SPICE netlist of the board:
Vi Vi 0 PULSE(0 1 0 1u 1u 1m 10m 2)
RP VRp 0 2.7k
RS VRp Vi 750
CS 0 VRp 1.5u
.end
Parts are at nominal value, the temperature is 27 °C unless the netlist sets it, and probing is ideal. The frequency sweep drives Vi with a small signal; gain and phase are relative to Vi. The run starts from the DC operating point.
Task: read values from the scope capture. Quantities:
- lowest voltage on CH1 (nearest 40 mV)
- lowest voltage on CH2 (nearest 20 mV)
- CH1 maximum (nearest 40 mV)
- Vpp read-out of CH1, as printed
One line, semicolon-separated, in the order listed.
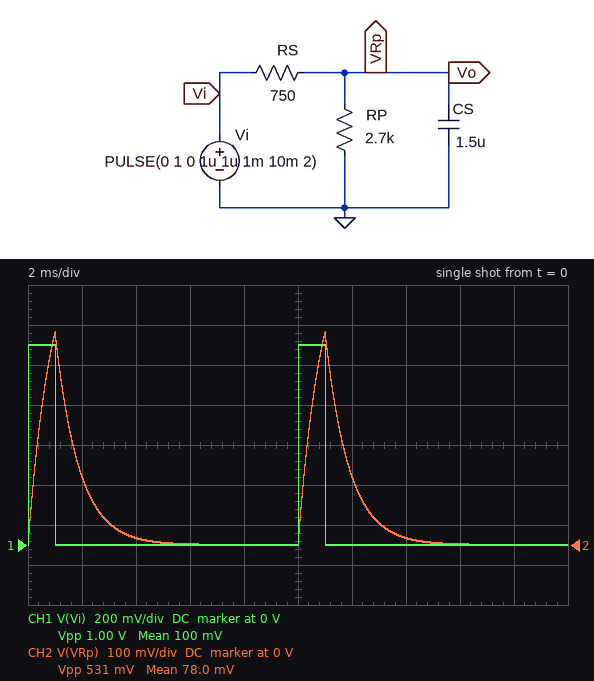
0 V; 0 V; 1.00 V; 1.00 V
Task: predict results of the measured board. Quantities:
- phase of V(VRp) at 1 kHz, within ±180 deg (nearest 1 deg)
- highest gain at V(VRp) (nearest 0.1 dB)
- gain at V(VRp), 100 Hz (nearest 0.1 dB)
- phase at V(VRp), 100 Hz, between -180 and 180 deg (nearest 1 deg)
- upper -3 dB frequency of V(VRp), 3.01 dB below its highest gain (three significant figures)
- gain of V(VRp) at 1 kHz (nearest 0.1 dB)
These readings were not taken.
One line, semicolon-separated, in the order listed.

-80 deg; -2.1 dB; -3.3 dB; -29 deg; 181 Hz; -17.1 dB
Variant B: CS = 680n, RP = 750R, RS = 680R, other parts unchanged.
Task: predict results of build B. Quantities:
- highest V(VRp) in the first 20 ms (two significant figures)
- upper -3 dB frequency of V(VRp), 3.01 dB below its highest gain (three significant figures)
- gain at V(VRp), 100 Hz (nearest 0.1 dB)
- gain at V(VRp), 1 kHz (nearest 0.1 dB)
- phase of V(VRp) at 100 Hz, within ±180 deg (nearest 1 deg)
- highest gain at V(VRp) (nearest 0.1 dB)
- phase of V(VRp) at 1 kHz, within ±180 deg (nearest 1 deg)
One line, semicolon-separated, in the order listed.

520 mV; 656 Hz; -5.7 dB; -10.8 dB; -9 deg; -5.6 dB; -57 deg
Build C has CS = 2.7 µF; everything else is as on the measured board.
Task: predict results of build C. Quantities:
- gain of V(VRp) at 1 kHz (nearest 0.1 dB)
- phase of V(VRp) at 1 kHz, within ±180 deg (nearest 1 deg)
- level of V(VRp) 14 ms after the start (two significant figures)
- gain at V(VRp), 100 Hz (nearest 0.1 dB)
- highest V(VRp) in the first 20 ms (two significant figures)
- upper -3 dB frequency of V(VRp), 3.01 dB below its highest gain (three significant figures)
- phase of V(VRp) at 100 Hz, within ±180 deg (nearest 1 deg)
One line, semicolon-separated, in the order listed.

-22.1 dB; -84 deg; 55 mV; -5.1 dB; 370 mV; 100 Hz; -45 deg
